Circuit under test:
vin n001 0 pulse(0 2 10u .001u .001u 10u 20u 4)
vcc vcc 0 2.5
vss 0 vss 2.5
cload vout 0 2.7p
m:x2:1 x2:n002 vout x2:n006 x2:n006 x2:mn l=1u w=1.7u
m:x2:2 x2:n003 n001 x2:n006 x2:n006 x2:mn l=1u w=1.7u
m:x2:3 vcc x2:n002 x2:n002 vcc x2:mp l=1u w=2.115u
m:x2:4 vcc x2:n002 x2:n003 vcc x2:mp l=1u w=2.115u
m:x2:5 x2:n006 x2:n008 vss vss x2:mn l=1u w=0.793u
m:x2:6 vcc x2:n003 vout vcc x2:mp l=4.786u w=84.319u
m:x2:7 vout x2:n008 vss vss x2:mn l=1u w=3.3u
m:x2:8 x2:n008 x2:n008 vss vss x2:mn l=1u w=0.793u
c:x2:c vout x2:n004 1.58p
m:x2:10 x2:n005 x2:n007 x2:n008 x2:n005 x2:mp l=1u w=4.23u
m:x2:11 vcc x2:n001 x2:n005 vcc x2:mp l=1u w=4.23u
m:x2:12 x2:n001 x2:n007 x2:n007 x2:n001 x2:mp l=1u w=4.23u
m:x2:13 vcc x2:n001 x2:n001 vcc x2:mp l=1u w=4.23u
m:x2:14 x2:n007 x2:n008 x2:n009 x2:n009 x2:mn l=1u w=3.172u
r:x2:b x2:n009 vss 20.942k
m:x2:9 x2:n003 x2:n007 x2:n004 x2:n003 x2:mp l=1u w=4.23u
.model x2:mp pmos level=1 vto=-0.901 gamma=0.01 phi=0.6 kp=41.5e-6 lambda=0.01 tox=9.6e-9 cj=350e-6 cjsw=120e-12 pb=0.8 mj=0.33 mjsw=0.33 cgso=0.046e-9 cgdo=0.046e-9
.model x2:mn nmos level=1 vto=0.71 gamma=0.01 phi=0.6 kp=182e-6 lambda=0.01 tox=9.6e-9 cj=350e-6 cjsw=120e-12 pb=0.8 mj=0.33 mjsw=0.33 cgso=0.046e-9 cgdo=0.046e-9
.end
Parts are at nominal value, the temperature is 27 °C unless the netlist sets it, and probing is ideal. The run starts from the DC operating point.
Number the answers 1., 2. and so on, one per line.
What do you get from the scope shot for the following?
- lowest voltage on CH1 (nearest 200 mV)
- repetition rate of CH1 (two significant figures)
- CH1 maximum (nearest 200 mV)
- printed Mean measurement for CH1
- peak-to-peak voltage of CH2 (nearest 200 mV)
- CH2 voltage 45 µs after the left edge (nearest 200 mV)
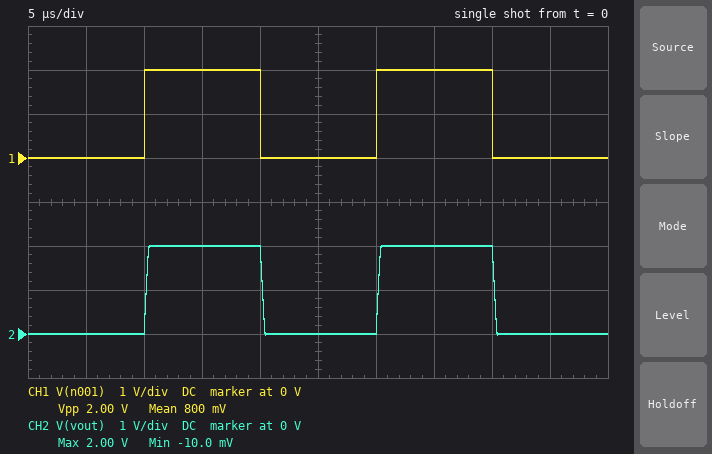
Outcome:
1. 0 V
2. 50 kHz
3. 2.0 V
4. 800 mV
5. 2.0 V
6. 0 V
